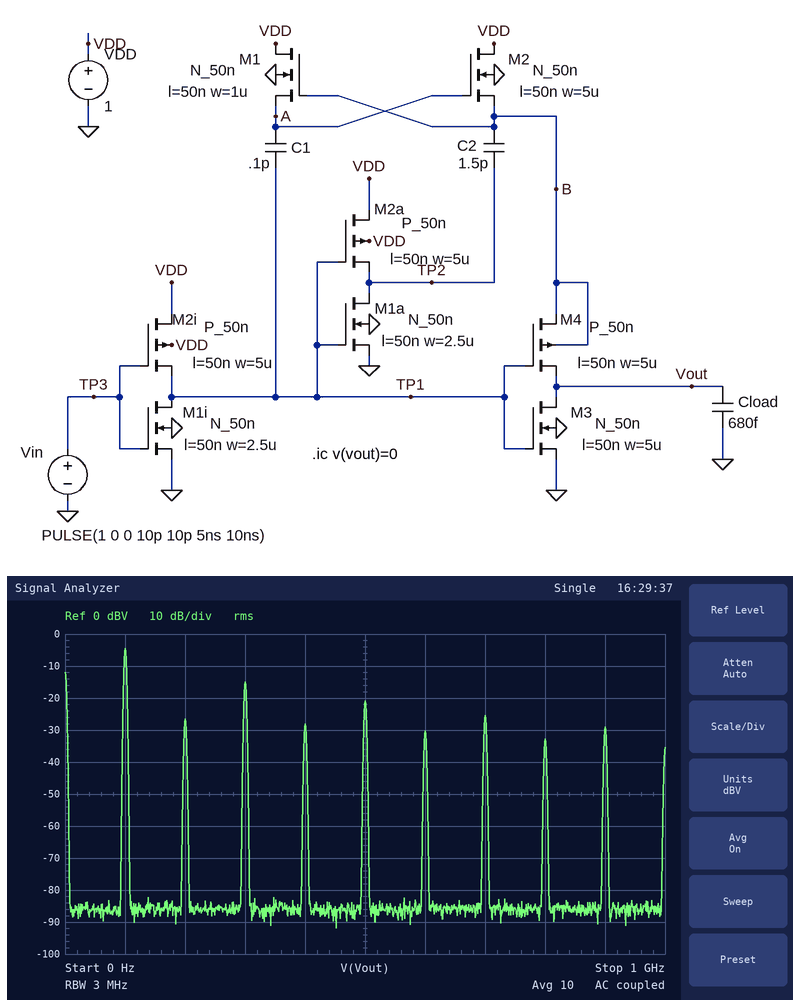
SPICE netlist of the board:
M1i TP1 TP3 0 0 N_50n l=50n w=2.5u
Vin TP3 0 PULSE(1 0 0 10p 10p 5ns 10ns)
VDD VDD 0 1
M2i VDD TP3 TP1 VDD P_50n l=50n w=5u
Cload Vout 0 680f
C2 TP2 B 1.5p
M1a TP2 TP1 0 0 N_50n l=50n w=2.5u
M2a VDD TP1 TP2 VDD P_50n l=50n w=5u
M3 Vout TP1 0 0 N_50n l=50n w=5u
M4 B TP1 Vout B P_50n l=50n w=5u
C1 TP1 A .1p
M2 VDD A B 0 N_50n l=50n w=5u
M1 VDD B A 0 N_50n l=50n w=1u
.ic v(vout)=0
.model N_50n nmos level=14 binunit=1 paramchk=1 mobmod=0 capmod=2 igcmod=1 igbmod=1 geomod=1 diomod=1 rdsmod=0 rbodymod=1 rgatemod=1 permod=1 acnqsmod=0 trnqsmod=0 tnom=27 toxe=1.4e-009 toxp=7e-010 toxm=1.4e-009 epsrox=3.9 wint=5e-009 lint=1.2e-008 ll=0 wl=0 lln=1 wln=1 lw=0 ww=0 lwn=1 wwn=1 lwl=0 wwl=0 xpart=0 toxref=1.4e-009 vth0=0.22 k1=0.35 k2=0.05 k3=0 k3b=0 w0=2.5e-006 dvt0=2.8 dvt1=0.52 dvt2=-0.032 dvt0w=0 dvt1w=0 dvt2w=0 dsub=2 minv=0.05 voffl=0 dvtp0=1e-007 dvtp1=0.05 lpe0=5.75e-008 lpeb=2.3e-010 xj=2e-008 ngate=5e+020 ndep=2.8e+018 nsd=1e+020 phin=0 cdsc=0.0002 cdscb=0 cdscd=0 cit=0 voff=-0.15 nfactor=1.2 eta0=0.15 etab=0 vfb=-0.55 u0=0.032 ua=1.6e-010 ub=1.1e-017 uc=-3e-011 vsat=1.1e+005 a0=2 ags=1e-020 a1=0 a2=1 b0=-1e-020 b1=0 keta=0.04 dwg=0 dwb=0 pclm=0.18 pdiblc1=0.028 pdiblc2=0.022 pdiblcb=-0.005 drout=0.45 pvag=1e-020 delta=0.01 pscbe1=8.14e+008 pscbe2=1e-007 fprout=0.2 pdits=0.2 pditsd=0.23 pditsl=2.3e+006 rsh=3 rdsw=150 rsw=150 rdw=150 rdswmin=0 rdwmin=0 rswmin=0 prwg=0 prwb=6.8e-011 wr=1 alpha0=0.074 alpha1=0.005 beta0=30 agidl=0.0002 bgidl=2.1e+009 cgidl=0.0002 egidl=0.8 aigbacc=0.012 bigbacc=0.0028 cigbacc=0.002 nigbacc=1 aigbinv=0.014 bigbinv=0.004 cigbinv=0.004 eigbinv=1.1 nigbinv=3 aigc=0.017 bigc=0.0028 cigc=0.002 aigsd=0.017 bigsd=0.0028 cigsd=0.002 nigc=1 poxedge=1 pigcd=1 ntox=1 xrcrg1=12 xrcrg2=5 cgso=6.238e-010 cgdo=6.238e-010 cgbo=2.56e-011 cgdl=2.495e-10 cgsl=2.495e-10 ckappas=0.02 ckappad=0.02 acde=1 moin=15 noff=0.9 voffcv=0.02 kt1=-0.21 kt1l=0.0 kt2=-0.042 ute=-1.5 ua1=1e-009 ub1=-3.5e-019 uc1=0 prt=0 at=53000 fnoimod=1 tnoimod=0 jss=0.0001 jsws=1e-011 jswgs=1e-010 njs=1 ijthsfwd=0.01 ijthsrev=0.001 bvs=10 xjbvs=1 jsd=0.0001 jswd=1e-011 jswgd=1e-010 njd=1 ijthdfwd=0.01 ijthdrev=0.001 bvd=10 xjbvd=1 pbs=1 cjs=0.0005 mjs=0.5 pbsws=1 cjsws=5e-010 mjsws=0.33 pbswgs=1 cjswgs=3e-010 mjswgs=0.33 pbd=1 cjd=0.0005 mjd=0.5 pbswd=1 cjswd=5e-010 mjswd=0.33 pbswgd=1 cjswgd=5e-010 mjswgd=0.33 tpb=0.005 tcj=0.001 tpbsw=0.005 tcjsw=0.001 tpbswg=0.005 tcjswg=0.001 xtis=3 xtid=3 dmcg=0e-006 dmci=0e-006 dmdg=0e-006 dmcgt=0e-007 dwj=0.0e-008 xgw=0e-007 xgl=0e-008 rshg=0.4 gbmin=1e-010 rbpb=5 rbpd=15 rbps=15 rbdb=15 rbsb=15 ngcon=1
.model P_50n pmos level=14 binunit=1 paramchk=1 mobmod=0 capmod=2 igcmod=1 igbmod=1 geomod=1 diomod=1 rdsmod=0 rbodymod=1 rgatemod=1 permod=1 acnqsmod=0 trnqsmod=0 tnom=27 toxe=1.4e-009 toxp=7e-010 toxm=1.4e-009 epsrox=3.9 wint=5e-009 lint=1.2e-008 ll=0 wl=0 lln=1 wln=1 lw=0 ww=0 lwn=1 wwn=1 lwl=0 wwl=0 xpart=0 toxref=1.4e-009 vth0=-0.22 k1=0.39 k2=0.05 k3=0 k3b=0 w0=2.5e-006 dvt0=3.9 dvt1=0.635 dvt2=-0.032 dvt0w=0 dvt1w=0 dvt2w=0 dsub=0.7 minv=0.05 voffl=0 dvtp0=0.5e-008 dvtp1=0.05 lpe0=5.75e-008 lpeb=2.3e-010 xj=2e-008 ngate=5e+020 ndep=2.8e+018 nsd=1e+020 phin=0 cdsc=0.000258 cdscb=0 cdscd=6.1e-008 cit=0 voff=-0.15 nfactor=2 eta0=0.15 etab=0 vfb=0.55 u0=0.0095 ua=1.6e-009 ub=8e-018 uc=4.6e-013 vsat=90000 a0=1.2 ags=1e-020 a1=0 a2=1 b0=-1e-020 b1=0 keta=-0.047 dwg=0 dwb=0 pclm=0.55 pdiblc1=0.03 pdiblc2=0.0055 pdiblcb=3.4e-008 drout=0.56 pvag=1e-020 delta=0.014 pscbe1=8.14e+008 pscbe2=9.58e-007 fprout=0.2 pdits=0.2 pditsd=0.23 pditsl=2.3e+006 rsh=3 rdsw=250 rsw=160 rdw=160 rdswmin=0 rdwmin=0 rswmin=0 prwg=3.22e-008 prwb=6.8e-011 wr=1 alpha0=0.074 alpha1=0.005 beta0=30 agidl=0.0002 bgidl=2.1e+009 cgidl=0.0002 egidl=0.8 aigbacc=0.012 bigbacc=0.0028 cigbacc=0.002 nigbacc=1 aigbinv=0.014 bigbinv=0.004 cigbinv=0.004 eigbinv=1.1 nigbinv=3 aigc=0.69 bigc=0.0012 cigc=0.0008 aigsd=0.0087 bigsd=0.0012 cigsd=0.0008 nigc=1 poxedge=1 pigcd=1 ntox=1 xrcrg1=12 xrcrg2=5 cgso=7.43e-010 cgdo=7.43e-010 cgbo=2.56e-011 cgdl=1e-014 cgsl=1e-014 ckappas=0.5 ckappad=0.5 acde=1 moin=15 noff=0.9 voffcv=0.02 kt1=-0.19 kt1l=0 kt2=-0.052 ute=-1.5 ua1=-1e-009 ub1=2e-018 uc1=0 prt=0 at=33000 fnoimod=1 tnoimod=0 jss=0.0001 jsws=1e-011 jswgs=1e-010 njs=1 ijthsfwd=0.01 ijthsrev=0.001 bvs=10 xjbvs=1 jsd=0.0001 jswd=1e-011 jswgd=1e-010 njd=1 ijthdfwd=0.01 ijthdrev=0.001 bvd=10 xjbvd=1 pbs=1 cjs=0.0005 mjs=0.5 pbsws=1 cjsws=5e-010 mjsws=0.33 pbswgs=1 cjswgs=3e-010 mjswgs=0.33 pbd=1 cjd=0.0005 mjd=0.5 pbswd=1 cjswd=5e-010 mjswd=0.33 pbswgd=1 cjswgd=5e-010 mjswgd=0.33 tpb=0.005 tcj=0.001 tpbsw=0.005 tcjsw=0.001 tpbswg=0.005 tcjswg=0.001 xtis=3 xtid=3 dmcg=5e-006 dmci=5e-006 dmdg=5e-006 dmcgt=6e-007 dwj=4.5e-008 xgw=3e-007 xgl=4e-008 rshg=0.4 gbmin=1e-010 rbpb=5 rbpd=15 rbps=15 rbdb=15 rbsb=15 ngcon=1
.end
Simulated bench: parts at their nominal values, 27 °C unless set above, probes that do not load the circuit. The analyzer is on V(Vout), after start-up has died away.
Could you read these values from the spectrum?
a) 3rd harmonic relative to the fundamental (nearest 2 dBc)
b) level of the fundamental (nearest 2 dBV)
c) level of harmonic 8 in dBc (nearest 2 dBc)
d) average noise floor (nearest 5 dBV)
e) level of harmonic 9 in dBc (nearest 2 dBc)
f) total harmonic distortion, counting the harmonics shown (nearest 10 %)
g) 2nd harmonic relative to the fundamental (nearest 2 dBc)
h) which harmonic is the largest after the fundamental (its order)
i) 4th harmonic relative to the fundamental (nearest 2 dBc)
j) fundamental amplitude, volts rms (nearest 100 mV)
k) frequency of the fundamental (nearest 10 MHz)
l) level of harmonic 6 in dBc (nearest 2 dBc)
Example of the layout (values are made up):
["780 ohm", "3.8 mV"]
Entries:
["-10 dBc", "-4 dBV", "-28 dBc", "-85 dBV", "-24 dBc", "40 %", "-22 dBc", "3", "-24 dBc", "600 mV", "100 MHz", "-26 dBc"]
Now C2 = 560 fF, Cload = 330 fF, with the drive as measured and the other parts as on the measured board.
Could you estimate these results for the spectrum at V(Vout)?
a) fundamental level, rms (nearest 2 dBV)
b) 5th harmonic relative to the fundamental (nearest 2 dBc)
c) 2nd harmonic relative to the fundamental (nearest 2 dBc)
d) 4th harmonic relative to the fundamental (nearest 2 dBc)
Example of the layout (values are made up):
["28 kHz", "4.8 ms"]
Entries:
["-6 dBV", "-14 dBc", "-28 dBc", "-28 dBc"]
